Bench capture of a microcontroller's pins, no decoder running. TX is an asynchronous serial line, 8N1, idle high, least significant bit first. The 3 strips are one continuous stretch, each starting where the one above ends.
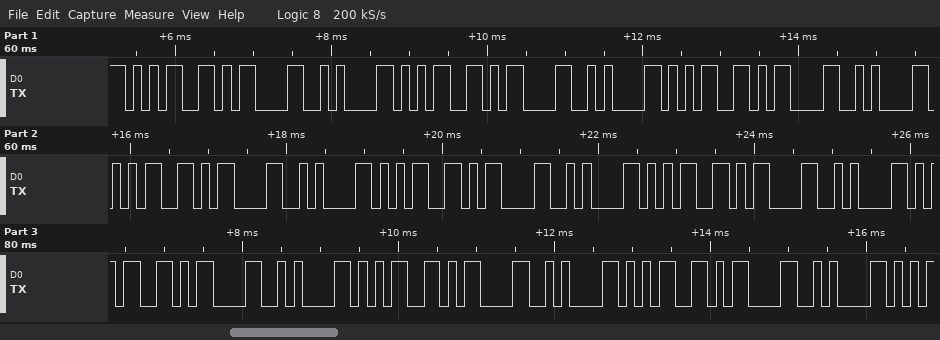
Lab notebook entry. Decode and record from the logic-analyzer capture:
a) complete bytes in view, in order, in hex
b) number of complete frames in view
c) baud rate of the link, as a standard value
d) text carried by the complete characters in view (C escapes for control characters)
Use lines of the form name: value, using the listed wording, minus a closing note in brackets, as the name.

complete bytes in view, in order, in hex: 0x35 0x0D 0x0A 0x35 0x0D 0x0A 0x35 0x0D 0x0A 0x35 0x0D 0x0A 0x35 0x0D 0x0A 0x35 0x0D 0x0A 0x35 0x0D 0x0A 0x35 0x0D 0x0A 0x35 0x0D 0x0A
number of complete frames in view: 27
baud rate of the link, as a standard value: 9600 baud
text carried by the complete characters in view: "5\r\n5\r\n5\r\n5\r\n5\r\n5\r\n5\r\n5\r\n5\r\n"
